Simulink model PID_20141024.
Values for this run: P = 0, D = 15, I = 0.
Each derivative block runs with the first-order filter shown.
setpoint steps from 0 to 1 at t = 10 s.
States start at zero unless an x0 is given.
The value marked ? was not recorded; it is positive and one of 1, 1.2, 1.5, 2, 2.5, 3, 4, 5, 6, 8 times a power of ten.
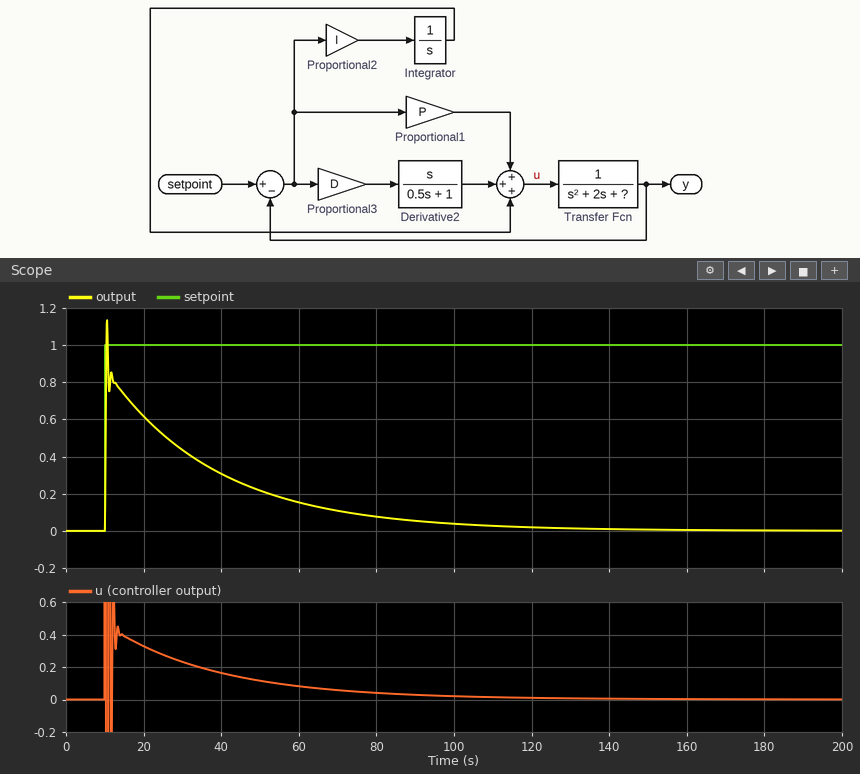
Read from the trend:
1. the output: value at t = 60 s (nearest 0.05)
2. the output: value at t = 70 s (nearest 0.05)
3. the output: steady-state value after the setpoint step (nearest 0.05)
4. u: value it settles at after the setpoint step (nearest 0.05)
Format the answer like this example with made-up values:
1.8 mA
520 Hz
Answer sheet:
0.15
0.10
0.00
0.00
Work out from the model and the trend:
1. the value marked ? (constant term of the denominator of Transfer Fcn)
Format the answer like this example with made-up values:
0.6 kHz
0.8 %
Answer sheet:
0.6
